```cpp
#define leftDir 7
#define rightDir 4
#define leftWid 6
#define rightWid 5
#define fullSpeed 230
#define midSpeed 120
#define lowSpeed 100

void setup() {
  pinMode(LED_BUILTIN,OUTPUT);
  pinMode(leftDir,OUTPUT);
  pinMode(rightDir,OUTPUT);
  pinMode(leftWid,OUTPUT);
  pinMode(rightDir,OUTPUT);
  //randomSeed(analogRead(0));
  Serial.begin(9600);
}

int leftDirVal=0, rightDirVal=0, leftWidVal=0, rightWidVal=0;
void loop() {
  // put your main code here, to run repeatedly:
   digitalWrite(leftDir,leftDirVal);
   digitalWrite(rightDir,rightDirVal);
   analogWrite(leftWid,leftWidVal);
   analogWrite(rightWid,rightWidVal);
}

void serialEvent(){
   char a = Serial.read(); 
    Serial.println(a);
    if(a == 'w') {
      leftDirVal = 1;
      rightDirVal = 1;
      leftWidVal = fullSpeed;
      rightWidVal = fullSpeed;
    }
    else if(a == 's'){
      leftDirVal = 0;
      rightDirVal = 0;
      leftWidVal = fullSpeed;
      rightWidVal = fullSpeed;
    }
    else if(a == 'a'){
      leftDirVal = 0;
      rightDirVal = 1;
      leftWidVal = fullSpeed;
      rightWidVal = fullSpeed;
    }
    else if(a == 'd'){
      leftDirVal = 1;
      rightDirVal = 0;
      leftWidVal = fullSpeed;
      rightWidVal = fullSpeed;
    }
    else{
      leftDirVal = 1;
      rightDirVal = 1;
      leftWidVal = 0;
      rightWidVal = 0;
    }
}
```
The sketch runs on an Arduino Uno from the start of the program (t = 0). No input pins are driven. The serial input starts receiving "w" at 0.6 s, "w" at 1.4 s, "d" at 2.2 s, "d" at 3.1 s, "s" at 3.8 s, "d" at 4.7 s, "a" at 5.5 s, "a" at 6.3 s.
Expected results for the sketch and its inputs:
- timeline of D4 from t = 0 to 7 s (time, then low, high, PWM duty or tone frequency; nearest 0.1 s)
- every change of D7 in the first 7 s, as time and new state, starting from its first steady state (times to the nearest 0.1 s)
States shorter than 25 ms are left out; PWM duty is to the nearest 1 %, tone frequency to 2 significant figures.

0 s low; 0.6 s high; 2.2 s low; 5.5 s high
0 s low; 0.6 s high; 3.8 s low; 4.7 s high; 5.5 s low
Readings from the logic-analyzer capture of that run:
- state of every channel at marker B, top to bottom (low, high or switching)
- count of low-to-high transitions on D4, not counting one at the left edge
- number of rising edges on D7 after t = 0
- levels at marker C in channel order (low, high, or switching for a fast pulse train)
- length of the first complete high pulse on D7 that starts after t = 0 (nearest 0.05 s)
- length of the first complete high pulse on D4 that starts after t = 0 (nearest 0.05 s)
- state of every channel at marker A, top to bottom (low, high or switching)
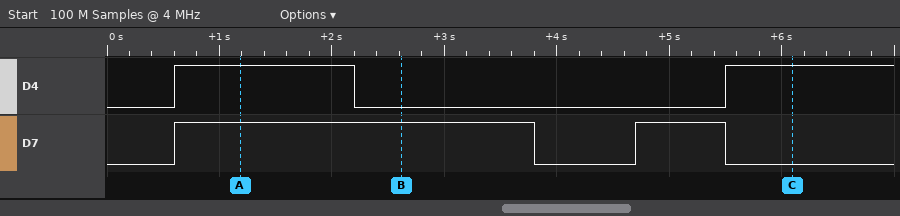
D4 low, D7 high
2
2
D4 high, D7 low
3.20 s
1.60 s
D4 high, D7 high
